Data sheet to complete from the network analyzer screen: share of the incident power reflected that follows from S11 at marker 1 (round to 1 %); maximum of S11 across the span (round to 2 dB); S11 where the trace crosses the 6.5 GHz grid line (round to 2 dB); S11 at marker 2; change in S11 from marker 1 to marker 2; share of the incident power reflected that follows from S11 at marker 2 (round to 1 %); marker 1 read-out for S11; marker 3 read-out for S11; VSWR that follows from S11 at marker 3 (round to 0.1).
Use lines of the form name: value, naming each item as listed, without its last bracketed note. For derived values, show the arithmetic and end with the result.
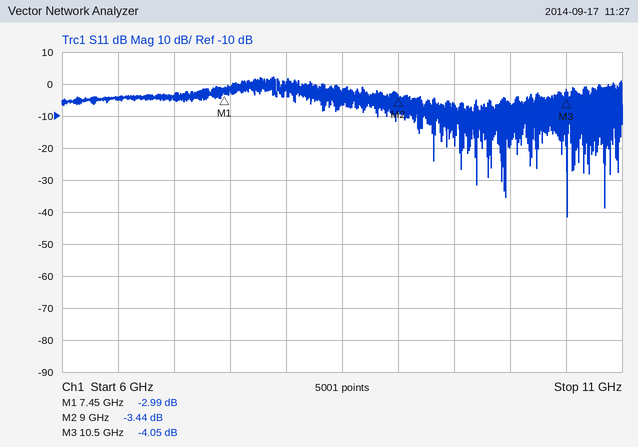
share of the incident power reflected that follows from S11 at marker 1: 10^(-2.99/10) ≈ 50 %
maximum of S11 across the span: 2 dB
S11 where the trace crosses the 6.5 GHz grid line: -4 dB
S11 at marker 2: -3.44 dB
change in S11 from marker 1 to marker 2: -3.44 − (-2.99) = -0.45 dB
share of the incident power reflected that follows from S11 at marker 2: 10^(-3.44/10) ≈ 45 %
marker 1 read-out for S11: -2.99 dB
marker 3 read-out for S11: -4.05 dB
VSWR that follows from S11 at marker 3: (1 + 0.6273)/(1 − 0.6273) ≈ 4.4
